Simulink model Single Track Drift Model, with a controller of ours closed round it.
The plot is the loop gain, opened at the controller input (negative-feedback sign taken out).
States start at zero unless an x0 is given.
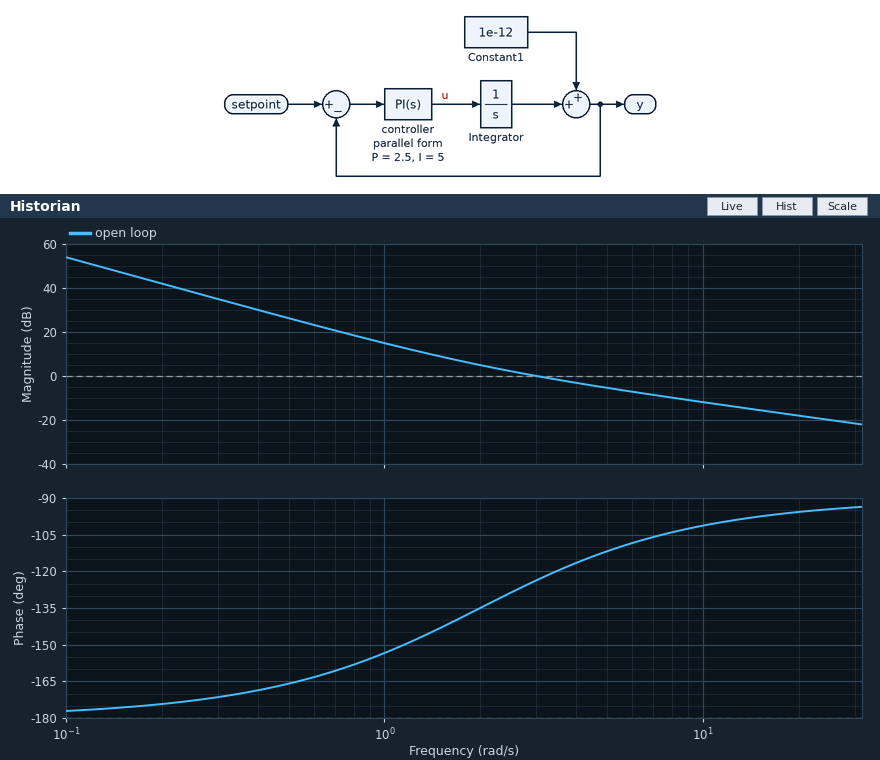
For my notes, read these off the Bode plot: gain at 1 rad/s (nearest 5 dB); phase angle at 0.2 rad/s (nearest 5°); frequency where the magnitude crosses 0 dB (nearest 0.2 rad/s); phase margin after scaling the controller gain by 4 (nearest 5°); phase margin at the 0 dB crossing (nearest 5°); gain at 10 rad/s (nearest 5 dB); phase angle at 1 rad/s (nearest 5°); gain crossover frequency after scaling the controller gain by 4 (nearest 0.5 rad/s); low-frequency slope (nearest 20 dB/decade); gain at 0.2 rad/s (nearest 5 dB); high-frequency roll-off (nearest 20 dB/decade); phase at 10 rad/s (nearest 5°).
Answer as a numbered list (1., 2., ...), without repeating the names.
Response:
1. 15 dB
2. -175°
3. 3.0 rad/s
4. 80°
5. 55°
6. -10 dB
7. -155°
8. 10.0 rad/s
9. -40 dB/decade
10. 40 dB
11. -20 dB/decade
12. -100°
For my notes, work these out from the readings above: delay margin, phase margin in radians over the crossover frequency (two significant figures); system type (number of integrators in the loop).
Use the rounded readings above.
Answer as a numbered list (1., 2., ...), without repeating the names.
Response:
1. 0.32 s
2. 2
